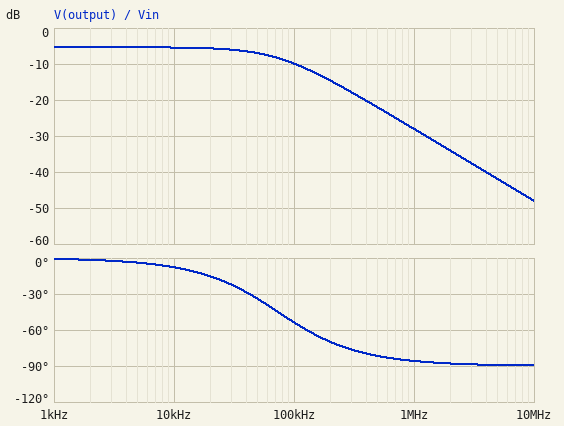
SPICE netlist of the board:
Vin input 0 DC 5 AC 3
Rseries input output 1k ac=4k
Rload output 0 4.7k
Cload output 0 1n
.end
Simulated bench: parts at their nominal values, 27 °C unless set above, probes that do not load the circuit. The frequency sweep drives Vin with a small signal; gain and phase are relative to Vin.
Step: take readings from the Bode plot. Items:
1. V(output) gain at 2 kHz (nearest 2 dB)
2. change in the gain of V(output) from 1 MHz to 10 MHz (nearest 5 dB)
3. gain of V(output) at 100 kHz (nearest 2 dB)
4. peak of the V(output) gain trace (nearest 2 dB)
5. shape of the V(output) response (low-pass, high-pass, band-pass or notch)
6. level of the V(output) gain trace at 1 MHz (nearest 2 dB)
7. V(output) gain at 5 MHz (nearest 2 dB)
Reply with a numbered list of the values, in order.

1. -6 dB
2. -20 dB
3. -10 dB
4. -6 dB
5. low-pass
6. -28 dB
7. -42 dB
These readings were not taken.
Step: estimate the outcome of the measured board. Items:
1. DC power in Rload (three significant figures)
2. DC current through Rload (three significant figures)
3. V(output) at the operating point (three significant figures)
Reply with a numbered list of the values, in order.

1. 3.62 mW
2. 877 µA
3. 4.12 V
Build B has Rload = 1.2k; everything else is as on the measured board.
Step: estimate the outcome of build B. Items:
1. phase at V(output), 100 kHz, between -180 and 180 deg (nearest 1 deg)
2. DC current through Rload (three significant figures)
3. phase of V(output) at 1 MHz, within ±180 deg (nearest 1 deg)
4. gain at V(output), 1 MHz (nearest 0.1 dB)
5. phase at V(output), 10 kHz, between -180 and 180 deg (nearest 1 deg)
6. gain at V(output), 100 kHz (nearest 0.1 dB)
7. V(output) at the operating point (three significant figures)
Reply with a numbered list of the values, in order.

1. -30 deg
2. 2.27 mA
3. -80 deg
4. -28.1 dB
5. -3 deg
6. -14.0 dB
7. 2.73 V
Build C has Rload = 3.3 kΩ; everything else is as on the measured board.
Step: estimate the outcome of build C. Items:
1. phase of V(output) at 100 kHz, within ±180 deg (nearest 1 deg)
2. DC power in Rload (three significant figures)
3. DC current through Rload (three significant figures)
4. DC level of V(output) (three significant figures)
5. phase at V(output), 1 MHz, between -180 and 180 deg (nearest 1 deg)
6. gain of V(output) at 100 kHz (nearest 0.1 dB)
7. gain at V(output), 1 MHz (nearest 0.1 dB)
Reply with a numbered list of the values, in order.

1. -49 deg
2. 4.46 mW
3. 1.16 mA
4. 3.84 V
5. -85 deg
6. -10.5 dB
7. -28.0 dB
